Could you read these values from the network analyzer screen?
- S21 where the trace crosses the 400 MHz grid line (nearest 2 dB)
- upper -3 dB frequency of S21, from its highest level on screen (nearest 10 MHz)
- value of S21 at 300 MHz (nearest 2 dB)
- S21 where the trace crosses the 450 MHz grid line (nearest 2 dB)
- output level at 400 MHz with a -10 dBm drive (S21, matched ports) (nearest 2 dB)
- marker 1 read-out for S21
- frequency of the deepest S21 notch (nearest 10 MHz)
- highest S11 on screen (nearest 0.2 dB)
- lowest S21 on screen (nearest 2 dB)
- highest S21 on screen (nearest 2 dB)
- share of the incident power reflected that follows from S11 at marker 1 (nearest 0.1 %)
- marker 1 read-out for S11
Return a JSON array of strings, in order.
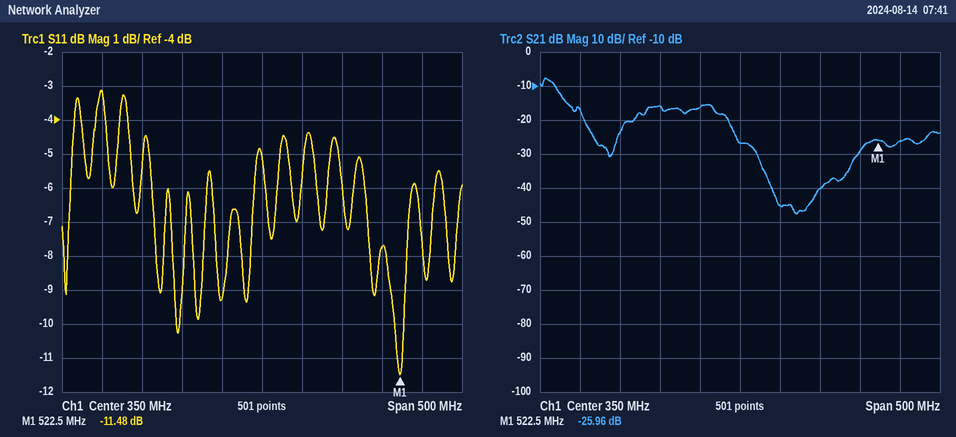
["-46 dB", "120 MHz", "-16 dB", "-40 dB", "-56 dBm", "-25.96 dB", "420 MHz", "-3.2 dB", "-48 dB", "-8 dB", "7.1 %", "-11.48 dB"]
